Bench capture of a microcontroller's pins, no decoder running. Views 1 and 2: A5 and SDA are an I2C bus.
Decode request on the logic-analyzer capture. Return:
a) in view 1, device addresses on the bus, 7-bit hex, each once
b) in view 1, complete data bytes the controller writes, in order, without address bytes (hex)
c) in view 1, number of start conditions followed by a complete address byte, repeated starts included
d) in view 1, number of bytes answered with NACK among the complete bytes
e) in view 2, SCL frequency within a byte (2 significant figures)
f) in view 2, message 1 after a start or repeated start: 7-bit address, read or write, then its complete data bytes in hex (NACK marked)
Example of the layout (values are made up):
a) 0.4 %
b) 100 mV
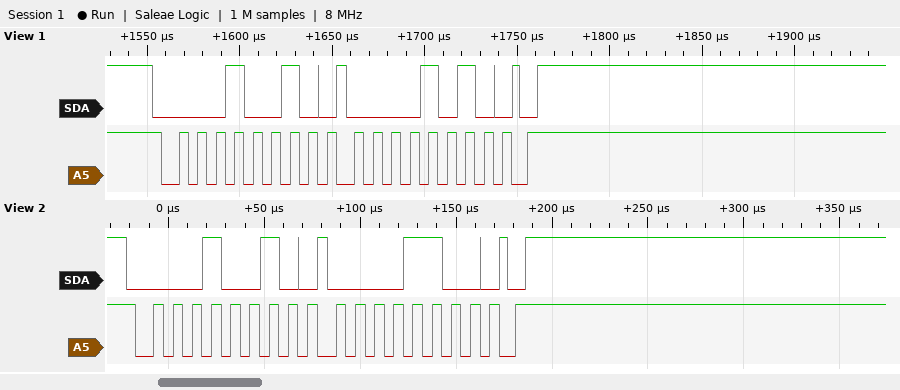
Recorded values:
a) 0x09
b) 0A
c) 1
d) 0
e) 100 kHz
f) 0x09 write: 0C
